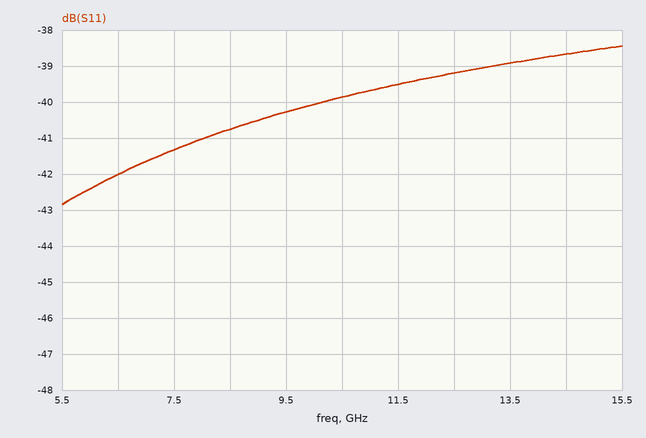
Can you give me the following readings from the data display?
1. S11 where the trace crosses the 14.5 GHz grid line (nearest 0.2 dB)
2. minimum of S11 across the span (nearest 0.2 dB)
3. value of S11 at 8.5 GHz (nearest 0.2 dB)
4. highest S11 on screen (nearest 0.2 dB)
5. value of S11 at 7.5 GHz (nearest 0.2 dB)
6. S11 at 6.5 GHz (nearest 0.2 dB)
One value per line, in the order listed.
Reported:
-38.6 dB
-42.8 dB
-40.8 dB
-38.4 dB
-41.4 dB
-42.0 dB
